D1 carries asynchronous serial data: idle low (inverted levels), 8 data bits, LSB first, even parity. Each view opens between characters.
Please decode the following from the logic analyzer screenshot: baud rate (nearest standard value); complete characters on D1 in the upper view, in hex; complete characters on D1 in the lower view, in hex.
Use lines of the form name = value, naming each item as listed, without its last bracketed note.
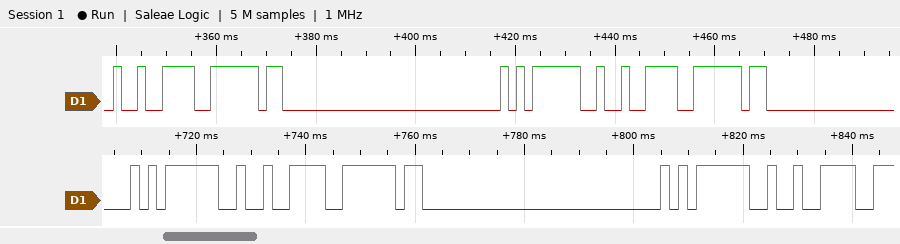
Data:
baud rate = 600 baud
complete characters on D1 in the upper view, in hex = 1B, 20, 05, 1B, 20
complete characters on D1 in the lower view, in hex = 05, 1B, 20, 05, 1B
